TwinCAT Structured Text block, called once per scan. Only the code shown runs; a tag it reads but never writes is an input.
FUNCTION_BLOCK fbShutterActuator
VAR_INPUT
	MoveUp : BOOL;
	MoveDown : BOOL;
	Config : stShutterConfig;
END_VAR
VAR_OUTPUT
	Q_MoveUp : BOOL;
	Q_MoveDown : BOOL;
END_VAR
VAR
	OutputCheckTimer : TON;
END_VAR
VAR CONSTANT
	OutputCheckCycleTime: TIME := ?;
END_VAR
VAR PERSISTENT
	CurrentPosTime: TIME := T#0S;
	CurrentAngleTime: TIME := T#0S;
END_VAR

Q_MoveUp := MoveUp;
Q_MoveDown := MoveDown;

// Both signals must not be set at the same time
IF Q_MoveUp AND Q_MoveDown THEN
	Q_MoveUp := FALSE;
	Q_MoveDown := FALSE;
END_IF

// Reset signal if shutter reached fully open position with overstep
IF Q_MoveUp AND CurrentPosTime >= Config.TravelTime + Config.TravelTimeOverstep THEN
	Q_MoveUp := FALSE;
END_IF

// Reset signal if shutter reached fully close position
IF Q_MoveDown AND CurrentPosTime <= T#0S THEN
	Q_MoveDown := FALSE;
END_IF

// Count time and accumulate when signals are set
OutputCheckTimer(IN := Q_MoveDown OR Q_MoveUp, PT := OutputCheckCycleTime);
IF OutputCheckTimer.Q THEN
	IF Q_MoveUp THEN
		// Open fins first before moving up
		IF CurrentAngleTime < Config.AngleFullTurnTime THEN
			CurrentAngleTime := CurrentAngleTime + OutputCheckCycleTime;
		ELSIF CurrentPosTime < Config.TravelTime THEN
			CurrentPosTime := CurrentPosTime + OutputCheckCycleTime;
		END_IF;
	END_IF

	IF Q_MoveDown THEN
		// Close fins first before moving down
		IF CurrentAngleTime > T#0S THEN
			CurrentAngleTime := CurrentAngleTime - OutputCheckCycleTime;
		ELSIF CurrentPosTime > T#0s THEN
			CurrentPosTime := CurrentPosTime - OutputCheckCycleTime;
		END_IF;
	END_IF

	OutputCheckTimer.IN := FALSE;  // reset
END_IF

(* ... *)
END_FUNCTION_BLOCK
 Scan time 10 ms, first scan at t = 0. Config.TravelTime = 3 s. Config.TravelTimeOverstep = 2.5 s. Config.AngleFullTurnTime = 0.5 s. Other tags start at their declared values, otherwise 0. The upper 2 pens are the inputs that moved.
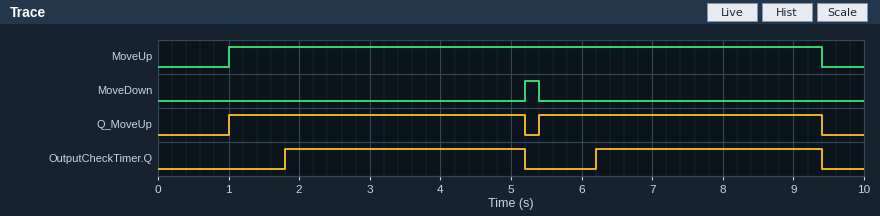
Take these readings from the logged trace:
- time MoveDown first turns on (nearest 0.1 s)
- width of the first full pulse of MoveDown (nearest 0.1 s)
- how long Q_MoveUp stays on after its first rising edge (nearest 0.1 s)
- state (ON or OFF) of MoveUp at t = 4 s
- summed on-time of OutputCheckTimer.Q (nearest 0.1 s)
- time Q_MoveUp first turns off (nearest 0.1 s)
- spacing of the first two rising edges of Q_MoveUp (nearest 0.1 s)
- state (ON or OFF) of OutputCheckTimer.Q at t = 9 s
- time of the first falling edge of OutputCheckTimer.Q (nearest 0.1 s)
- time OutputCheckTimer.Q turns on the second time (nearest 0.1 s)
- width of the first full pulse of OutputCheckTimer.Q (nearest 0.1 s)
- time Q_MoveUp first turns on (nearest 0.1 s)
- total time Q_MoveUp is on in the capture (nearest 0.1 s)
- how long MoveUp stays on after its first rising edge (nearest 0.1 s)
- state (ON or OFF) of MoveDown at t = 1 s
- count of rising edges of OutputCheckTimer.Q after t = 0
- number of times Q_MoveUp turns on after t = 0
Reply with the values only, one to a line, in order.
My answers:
5.2 s
0.2 s
4.2 s
ON
6.6 s
5.2 s
4.4 s
ON
5.2 s
6.2 s
3.4 s
1.0 s
8.2 s
8.4 s
OFF
2
2
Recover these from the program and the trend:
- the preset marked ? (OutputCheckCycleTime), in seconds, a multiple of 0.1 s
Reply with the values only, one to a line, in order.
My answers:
0.8 s
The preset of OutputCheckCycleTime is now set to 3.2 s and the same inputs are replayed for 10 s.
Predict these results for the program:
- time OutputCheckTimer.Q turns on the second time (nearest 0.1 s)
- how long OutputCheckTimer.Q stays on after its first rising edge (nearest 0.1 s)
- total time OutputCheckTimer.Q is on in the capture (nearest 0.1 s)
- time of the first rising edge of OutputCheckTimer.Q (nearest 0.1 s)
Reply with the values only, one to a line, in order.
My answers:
8.6 s
1.0 s
1.8 s
4.2 s
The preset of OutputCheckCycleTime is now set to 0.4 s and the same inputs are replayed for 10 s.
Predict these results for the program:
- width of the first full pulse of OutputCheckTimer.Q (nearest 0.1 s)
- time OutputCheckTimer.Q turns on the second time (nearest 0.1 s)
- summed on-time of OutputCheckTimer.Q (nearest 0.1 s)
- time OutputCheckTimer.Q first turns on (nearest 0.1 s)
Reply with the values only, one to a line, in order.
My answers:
3.8 s
5.8 s
7.4 s
1.4 s
